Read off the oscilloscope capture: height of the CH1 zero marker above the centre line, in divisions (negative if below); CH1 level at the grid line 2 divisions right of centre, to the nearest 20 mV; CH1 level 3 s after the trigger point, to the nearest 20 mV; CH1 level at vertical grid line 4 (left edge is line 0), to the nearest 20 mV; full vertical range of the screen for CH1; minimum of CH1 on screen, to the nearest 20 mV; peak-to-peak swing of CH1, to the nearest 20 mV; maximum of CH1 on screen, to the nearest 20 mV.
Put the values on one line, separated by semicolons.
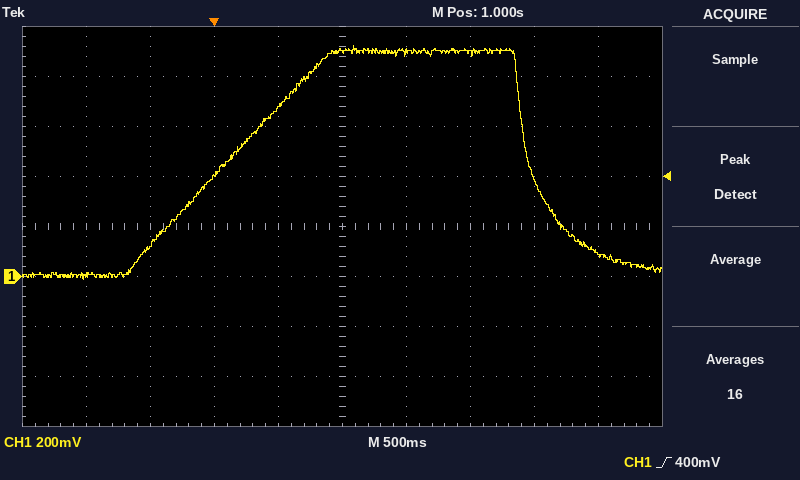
-1.0 div; 900 mV; 100 mV; 680 mV; 1.6 V; -20 mV; 940 mV; 920 mV
